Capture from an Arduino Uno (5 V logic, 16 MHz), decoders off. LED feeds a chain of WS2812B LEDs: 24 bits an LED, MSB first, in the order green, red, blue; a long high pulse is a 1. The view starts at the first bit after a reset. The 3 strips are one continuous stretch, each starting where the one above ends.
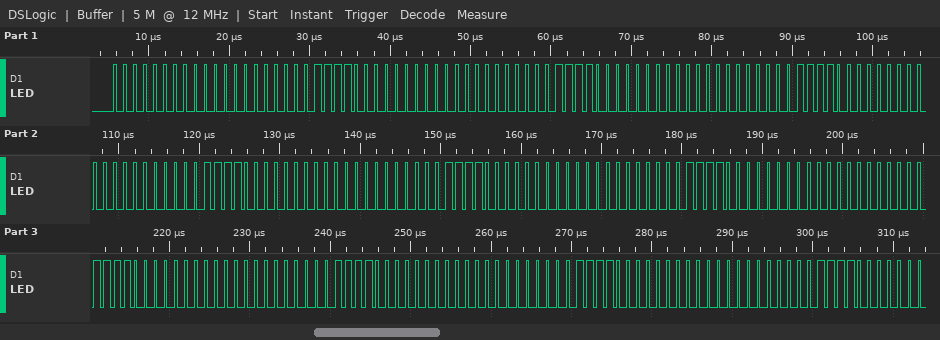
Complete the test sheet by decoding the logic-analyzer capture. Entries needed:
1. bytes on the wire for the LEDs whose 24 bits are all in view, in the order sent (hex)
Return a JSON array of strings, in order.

["00 00 0F 00 00 0F 00 00 0F 00 00 0F 00 00 0F 00 00 0F 00 00 0F 00 00 0F 00 00 0F 00 00 0F"]
